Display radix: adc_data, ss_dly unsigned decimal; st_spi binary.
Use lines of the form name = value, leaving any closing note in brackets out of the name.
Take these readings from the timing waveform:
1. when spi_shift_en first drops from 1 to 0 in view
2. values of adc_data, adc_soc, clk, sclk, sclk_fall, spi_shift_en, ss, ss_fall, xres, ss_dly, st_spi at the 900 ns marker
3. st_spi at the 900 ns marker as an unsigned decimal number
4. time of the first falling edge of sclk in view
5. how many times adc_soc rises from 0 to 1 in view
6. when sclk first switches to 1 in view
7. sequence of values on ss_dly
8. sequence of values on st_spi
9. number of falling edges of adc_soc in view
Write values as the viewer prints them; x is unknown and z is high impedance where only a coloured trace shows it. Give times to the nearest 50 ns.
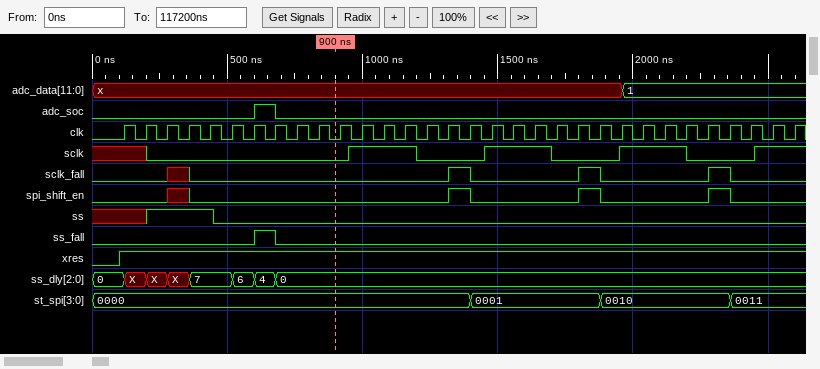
when spi_shift_en first drops from 1 to 0 in view = 1400 ns
values of adc_data, adc_soc, clk, sclk, sclk_fall, spi_shift_en, ss, ss_fall, xres, ss_dly, st_spi at the 900 ns marker = adc_data=x, adc_soc=0, clk=0, sclk=0, sclk_fall=0, spi_shift_en=0, ss=0, ss_fall=0, xres=1, ss_dly=0, st_spi=0000
st_spi at the 900 ns marker as an unsigned decimal number = 0
time of the first falling edge of sclk in view = 1200 ns
how many times adc_soc rises from 0 to 1 in view = 1
when sclk first switches to 1 in view = 950 ns
sequence of values on ss_dly = 0, X, X, X, 7, 6, 4, 0
sequence of values on st_spi = 0000, 0001, 0010, 0011
number of falling edges of adc_soc in view = 1
